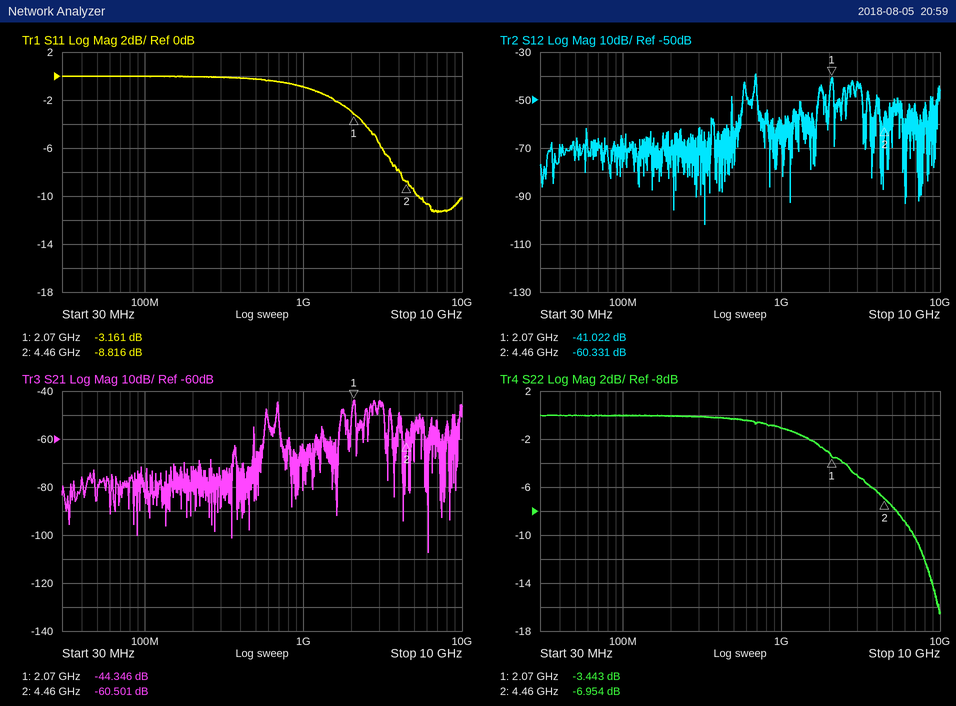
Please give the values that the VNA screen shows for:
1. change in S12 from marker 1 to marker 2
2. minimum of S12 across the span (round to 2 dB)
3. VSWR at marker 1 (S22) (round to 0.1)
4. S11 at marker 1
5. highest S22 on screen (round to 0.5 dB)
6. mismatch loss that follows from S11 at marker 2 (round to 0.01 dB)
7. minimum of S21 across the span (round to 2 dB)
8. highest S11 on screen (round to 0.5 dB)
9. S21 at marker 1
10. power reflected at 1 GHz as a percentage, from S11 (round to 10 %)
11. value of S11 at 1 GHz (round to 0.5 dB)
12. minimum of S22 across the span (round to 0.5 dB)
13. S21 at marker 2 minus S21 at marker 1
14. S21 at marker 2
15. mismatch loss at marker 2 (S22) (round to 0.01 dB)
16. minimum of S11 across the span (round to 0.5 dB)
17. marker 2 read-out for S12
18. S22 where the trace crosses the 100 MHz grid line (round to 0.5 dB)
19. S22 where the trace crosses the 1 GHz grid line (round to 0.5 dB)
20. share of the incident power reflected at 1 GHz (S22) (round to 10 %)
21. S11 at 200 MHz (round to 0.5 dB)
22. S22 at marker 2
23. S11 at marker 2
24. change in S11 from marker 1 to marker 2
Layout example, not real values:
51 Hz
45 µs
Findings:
-19.309 dB
-102 dB
5.1
-3.161 dB
0.0 dB
0.61 dB
-108 dB
0.0 dB
-44.346 dB
80 %
-1.0 dB
-16.5 dB
-16.155 dB
-60.501 dB
0.98 dB
-11.5 dB
-60.331 dB
0.0 dB
-1.0 dB
80 %
0.0 dB
-6.954 dB
-8.816 dB
-5.655 dB
